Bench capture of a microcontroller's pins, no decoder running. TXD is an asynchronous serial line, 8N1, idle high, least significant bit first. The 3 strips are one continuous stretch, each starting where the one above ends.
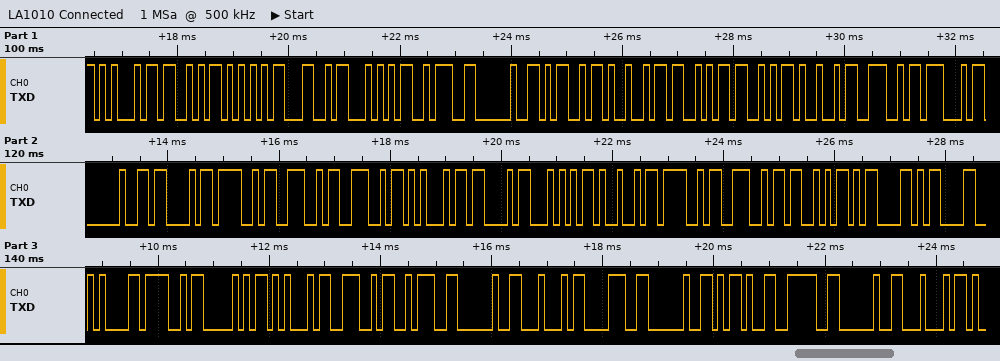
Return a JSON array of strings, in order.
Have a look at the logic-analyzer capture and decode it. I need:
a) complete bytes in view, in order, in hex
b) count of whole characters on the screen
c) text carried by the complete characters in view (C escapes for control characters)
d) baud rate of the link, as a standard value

["45 53 55 4C 54 3A 20 4D 49 53 53 49 4E 47 20 43 4F 4E 4E 45 43 54 49 4F 4E 53 0D 0D 0A 4F 50 45 4E 3A 20 44 38 20 2D 3E 20 44", "42", "\"ESULT: MISSING CONNECTIONS\\r\\r\\nOPEN: D8 -> D\"", "9600 baud"]
